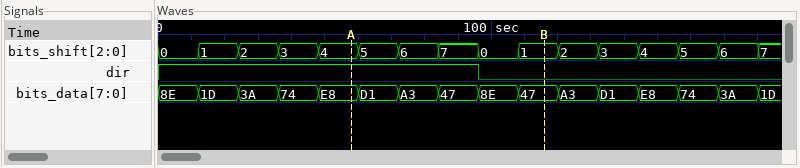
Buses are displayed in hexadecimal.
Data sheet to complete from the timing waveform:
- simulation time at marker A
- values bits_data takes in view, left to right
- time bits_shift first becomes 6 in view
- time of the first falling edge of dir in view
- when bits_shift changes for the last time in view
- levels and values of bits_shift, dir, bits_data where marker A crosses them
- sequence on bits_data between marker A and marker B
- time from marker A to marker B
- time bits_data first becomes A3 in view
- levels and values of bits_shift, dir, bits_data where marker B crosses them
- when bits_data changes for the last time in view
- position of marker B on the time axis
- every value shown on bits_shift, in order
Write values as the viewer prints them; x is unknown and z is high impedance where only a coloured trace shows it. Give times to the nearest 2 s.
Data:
58 s
8E, 1D, 3A, 74, E8, D1, A3, 47, 8E, 47, A3, D1, E8, 74, 3A, 1D
72 s
96 s
180 s
bits_shift=4, dir=1, bits_data=E8
E8, D1, A3, 47, 8E, 47
58 s
72 s
bits_shift=1, dir=0, bits_data=47
180 s
116 s
0, 1, 2, 3, 4, 5, 6, 7, 0, 1, 2, 3, 4, 5, 6, 7
